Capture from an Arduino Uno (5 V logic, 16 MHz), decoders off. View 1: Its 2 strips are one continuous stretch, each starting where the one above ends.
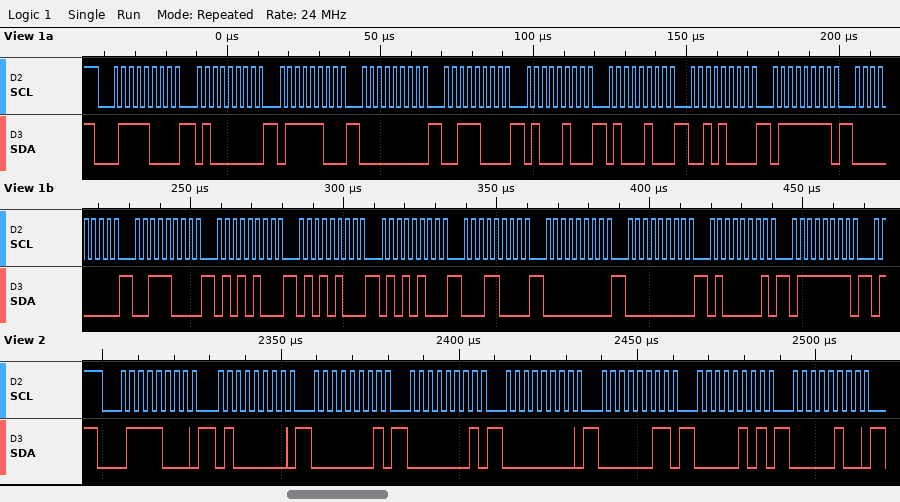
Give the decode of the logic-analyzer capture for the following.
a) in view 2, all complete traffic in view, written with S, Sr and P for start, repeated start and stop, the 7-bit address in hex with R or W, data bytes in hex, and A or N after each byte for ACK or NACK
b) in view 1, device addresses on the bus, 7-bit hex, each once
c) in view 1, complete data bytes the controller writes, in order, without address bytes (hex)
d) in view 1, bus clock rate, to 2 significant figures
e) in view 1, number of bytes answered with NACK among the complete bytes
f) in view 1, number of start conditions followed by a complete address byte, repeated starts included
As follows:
S 3CW A 40 A 01 A 01 A 00 A 03 A 05 A 04 A
0x3C
40 7C 00 38 44 44 28 7F 00 38 54 54 54 18 00 00 41 7F
400 kHz
0
1
